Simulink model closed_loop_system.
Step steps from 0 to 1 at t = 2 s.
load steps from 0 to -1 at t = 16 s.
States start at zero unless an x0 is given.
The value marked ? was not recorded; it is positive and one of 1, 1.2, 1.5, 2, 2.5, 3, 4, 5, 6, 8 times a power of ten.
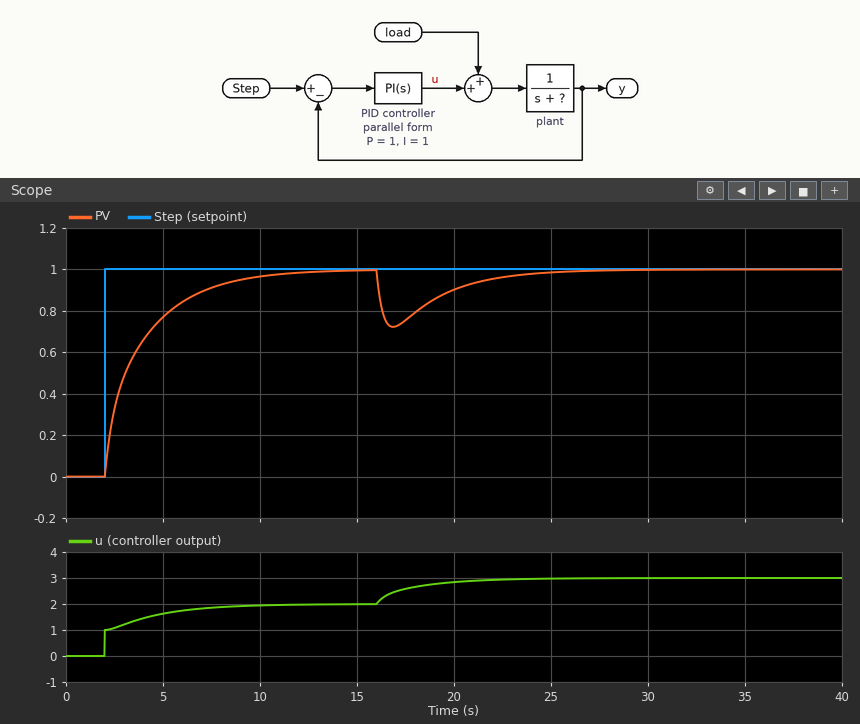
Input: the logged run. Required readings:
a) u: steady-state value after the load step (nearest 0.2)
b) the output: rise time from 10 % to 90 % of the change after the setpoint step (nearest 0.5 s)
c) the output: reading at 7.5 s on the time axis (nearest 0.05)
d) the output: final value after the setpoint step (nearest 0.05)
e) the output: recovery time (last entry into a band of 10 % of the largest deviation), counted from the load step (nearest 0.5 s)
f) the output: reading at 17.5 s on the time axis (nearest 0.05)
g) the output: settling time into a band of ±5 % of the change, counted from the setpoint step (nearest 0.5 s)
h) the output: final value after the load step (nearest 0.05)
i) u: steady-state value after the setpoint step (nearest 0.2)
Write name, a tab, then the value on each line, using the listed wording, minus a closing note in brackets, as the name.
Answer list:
u: steady-state value after the load step	3.0
the output: rise time from 10 % to 90 % of the change after the setpoint step	5.0 s
the output: reading at 7.5 s on the time axis	0.90
the output: final value after the setpoint step	1.00
the output: recovery time (last entry into a band of 10 % of the largest deviation), counted from the load step	7.5 s
the output: reading at 17.5 s on the time axis	0.75
the output: settling time into a band of ±5 % of the change, counted from the setpoint step	7.0 s
the output: final value after the load step	1.00
u: steady-state value after the setpoint step	2.0
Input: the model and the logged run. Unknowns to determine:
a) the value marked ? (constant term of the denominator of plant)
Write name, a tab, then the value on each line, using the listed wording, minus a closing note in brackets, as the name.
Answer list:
the value marked ?	2
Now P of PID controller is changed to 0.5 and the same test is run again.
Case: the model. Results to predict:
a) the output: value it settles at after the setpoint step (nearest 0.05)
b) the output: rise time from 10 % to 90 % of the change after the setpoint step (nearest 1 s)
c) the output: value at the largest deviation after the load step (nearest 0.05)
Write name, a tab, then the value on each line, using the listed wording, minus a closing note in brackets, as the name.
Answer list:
the output: value it settles at after the setpoint step	1.00
the output: rise time from 10 % to 90 % of the change after the setpoint step	4 s
the output: value at the largest deviation after the load step	0.70
